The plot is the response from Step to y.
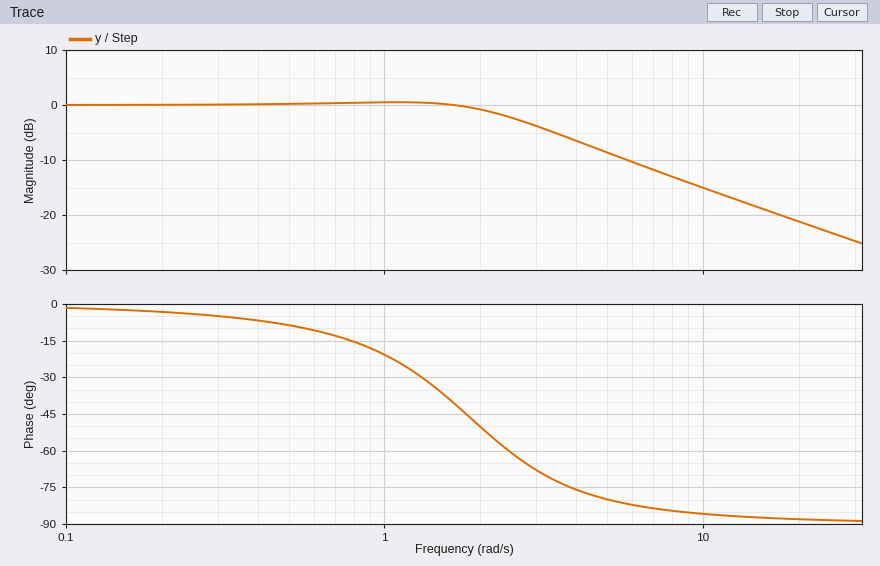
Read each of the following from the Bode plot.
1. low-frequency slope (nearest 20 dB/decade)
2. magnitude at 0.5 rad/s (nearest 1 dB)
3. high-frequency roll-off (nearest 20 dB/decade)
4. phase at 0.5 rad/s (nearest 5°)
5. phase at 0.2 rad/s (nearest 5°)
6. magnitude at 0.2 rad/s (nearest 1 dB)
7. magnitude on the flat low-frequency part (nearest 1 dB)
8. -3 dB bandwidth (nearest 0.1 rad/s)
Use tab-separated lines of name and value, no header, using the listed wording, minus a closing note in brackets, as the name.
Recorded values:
low-frequency slope	0 dB/decade
magnitude at 0.5 rad/s	0 dB
high-frequency roll-off	-20 dB/decade
phase at 0.5 rad/s	-10°
phase at 0.2 rad/s	-5°
magnitude at 0.2 rad/s	0 dB
magnitude on the flat low-frequency part	0 dB
-3 dB bandwidth	2.7 rad/s
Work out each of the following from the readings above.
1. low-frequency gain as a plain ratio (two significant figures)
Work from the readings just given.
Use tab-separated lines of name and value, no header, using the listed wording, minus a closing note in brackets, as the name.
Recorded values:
low-frequency gain as a plain ratio	1.0
